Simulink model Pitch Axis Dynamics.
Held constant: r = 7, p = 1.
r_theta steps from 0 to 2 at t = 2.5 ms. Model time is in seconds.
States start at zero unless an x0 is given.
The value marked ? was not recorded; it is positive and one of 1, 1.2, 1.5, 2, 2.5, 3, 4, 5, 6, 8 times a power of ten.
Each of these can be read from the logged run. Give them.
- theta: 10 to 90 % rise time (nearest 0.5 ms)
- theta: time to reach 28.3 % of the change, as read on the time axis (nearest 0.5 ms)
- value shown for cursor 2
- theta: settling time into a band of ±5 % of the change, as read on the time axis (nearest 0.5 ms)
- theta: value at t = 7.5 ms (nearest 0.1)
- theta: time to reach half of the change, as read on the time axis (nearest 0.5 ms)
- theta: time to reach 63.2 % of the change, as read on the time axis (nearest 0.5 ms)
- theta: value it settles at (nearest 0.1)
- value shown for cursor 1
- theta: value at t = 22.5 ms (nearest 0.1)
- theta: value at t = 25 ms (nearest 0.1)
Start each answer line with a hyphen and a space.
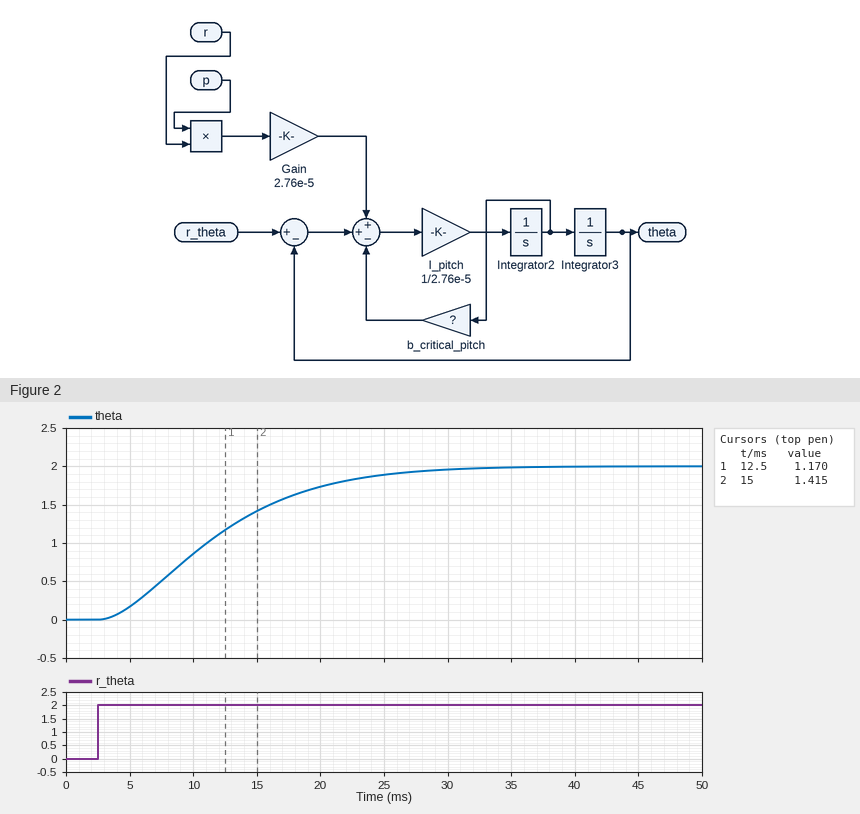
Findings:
- 16.5 ms
- 8.0 ms
- 1.415
- 25.5 ms
- 0.5
- 11.0 ms
- 13.5 ms
- 2.0
- 1.170
- 1.8
- 1.9
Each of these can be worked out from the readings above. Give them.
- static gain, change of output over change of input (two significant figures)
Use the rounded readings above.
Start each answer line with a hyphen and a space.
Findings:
- 1.0
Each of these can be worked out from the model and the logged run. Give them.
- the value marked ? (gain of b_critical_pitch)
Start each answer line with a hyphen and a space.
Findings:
- 0.01
